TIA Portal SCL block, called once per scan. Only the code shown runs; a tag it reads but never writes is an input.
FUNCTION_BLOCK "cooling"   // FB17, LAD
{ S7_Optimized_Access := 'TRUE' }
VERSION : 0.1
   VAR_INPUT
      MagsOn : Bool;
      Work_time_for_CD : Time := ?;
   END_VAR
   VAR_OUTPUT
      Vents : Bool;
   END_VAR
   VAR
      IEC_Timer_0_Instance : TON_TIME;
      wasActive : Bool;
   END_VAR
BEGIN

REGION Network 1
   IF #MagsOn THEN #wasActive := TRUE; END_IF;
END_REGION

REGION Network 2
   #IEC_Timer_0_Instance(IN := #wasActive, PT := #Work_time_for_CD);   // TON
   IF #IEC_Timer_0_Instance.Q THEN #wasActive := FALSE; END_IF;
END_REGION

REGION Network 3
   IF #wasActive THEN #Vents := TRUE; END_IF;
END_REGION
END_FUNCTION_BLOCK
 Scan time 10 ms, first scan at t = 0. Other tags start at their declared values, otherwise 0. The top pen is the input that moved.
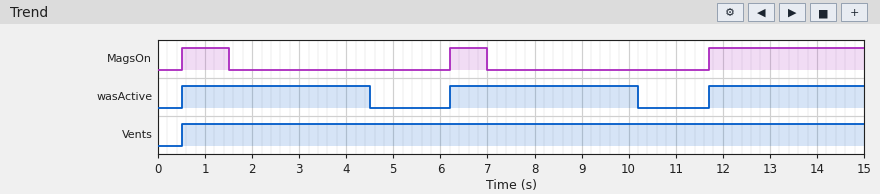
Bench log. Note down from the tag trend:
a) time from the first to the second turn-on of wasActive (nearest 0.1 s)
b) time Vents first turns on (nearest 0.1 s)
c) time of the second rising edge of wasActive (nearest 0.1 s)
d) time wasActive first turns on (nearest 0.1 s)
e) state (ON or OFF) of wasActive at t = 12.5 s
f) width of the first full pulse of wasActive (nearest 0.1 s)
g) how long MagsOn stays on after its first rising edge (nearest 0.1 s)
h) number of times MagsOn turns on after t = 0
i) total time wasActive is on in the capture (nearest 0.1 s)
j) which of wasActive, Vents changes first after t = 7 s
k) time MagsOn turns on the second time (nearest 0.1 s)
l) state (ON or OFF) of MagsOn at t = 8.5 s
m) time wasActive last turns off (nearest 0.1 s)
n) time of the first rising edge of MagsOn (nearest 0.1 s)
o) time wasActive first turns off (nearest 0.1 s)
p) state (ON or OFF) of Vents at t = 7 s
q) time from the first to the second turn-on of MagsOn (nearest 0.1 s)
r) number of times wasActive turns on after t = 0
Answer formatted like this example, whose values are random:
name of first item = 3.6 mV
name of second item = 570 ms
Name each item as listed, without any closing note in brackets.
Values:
time from the first to the second turn-on of wasActive = 5.7 s
time Vents first turns on = 0.5 s
time of the second rising edge of wasActive = 6.2 s
time wasActive first turns on = 0.5 s
state (ON or OFF) of wasActive at t = 12.5 s = ON
width of the first full pulse of wasActive = 4.0 s
how long MagsOn stays on after its first rising edge = 1.0 s
number of times MagsOn turns on after t = 0 = 3
total time wasActive is on in the capture = 11.3 s
which of wasActive, Vents changes first after t = 7 s = wasActive
time MagsOn turns on the second time = 6.2 s
state (ON or OFF) of MagsOn at t = 8.5 s = OFF
time wasActive last turns off = 10.2 s
time of the first rising edge of MagsOn = 0.5 s
time wasActive first turns off = 4.5 s
state (ON or OFF) of Vents at t = 7 s = ON
time from the first to the second turn-on of MagsOn = 5.7 s
number of times wasActive turns on after t = 0 = 3
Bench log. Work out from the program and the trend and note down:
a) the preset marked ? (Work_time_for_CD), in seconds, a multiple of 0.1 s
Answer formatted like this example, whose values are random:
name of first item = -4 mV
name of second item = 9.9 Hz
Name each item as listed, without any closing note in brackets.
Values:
the preset marked ? (Work_time_for_CD), in seconds, a multiple of 0.1 s = 4.0 s
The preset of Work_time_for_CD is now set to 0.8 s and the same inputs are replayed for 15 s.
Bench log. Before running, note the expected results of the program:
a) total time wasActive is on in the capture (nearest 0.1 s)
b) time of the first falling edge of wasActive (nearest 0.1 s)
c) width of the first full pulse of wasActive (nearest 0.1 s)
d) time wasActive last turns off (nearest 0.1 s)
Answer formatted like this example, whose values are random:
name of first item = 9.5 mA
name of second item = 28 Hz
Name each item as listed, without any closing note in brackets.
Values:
total time wasActive is on in the capture = 2.4 s
time of the first falling edge of wasActive = 1.3 s
width of the first full pulse of wasActive = 0.8 s
time wasActive last turns off = 12.5 s
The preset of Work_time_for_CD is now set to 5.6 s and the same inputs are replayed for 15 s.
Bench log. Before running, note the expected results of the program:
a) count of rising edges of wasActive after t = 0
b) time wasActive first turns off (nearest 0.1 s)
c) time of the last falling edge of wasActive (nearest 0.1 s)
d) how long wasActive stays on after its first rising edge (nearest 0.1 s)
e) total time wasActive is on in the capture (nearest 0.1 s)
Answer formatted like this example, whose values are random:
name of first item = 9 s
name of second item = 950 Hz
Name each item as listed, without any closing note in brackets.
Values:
count of rising edges of wasActive after t = 0 = 2
time wasActive first turns off = 6.1 s
time of the last falling edge of wasActive = 11.8 s
how long wasActive stays on after its first rising edge = 5.6 s
total time wasActive is on in the capture = 11.2 s
